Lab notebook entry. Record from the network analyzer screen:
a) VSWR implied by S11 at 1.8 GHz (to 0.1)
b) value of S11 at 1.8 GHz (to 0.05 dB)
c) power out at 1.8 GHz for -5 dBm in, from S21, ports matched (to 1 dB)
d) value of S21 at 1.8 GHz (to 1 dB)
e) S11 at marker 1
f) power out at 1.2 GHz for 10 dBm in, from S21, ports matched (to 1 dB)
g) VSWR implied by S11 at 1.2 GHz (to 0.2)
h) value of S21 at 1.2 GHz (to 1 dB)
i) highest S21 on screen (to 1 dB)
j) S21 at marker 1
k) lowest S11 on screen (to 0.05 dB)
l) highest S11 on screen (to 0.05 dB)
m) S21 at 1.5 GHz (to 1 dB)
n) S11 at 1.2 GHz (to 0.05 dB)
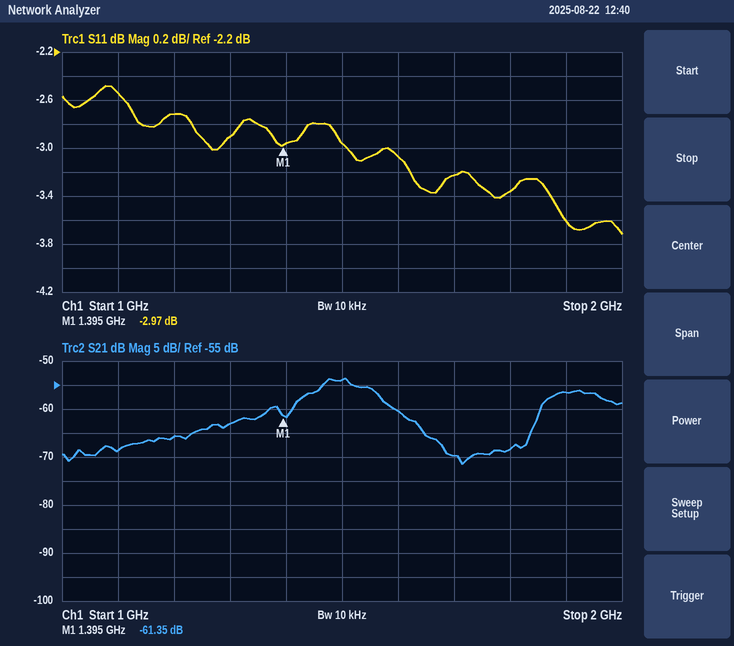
5.2
-3.35 dB
-73 dBm
-68 dB
-2.97 dB
-56 dBm
6.4
-66 dB
-54 dB
-61.35 dB
-3.70 dB
-2.50 dB
-54 dB
-2.70 dB
